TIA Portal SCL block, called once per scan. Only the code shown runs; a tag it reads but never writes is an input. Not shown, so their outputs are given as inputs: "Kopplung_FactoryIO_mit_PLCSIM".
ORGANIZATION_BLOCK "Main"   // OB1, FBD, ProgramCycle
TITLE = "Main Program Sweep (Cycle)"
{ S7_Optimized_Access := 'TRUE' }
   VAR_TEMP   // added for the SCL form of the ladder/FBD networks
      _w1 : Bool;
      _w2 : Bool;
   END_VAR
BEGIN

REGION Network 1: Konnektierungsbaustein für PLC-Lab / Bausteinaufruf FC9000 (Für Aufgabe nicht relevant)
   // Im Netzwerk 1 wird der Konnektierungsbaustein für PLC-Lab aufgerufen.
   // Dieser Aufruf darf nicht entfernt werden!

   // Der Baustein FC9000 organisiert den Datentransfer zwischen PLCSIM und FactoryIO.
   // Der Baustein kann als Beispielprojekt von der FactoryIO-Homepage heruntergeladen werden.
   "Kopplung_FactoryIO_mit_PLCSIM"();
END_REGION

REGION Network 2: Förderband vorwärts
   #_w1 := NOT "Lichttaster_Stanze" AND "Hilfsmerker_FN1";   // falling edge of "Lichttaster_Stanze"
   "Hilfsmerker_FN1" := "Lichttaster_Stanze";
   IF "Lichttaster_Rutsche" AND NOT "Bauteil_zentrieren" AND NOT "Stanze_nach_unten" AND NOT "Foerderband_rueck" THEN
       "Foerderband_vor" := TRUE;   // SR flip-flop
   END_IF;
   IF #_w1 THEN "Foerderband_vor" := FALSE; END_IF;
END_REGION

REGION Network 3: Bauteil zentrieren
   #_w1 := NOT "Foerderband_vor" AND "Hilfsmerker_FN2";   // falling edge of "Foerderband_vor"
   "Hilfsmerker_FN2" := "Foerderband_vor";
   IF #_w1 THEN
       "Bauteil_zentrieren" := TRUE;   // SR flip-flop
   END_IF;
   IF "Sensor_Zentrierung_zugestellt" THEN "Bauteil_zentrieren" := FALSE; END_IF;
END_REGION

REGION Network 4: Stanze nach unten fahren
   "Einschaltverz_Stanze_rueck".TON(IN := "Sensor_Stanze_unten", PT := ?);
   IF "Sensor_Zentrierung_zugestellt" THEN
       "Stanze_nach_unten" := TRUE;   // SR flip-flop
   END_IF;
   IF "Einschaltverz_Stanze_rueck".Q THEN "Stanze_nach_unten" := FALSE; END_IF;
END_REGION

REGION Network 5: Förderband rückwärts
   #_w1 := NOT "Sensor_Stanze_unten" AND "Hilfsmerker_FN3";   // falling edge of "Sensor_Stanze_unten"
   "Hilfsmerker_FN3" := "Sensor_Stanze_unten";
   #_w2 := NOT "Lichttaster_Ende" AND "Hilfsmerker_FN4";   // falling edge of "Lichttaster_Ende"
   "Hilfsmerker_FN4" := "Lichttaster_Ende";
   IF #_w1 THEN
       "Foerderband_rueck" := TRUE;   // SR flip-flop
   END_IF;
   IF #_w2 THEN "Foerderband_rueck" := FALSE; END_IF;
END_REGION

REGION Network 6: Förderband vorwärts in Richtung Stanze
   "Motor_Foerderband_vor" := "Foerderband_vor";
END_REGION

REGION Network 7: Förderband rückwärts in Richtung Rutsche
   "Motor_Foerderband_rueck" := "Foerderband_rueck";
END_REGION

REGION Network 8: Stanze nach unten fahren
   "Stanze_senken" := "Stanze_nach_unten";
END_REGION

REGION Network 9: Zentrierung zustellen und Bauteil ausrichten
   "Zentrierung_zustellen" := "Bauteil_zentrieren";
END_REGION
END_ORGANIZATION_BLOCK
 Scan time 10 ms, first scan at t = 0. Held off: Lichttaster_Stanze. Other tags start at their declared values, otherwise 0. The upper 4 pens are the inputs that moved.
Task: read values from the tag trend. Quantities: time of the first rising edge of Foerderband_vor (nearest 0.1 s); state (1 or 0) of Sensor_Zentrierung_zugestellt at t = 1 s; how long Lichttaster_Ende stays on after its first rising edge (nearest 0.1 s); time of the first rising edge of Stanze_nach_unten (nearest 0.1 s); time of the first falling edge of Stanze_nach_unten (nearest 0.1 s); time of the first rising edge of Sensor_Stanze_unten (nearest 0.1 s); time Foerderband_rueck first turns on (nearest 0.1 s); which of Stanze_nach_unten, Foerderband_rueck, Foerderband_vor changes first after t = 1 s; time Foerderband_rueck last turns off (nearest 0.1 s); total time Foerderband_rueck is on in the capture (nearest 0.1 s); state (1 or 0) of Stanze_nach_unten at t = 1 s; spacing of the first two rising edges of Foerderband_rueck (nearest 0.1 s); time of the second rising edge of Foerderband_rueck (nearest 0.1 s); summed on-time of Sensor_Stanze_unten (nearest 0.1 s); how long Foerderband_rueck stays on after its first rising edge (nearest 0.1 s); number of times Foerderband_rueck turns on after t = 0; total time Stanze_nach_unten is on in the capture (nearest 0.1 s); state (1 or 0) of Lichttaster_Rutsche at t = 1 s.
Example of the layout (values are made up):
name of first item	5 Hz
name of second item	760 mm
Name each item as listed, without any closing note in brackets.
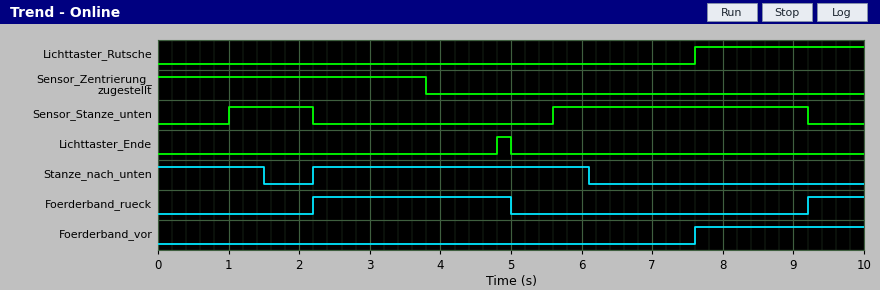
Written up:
time of the first rising edge of Foerderband_vor	7.6 s
state (1 or 0) of Sensor_Zentrierung_zugestellt at t = 1 s	1
how long Lichttaster_Ende stays on after its first rising edge	0.2 s
time of the first rising edge of Stanze_nach_unten	2.2 s
time of the first falling edge of Stanze_nach_unten	1.5 s
time of the first rising edge of Sensor_Stanze_unten	1.0 s
time Foerderband_rueck first turns on	2.2 s
which of Stanze_nach_unten, Foerderband_rueck, Foerderband_vor changes first after t = 1 s	Stanze_nach_unten
time Foerderband_rueck last turns off	5.0 s
total time Foerderband_rueck is on in the capture	3.6 s
state (1 or 0) of Stanze_nach_unten at t = 1 s	1
spacing of the first two rising edges of Foerderband_rueck	7.0 s
time of the second rising edge of Foerderband_rueck	9.2 s
summed on-time of Sensor_Stanze_unten	4.8 s
how long Foerderband_rueck stays on after its first rising edge	2.8 s
number of times Foerderband_rueck turns on after t = 0	2
total time Stanze_nach_unten is on in the capture	5.4 s
state (1 or 0) of Lichttaster_Rutsche at t = 1 s	0
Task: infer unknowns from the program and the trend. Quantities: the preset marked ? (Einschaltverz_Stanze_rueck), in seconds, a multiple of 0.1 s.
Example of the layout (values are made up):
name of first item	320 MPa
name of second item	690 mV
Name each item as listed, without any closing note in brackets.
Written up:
the preset marked ? (Einschaltverz_Stanze_rueck), in seconds, a multiple of 0.1 s	0.5 s
